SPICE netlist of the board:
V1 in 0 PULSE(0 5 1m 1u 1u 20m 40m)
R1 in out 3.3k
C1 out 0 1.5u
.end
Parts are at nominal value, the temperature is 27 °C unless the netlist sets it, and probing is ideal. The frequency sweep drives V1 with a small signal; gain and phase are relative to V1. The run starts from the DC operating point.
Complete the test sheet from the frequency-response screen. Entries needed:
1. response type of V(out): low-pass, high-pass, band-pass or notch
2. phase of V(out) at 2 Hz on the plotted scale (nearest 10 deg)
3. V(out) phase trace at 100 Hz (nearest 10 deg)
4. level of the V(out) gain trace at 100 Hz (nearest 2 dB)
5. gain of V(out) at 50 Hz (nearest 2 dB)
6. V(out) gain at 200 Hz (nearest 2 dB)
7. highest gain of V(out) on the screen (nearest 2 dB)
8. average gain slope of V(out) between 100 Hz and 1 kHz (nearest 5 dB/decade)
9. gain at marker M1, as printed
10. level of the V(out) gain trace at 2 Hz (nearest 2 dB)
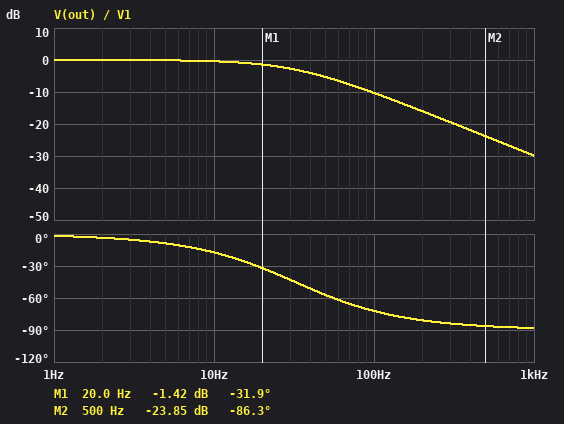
low-pass
0 deg
-70 deg
-10 dB
-6 dB
-16 dB
0 dB
-20 dB/decade
-1.42 dB
0 dB
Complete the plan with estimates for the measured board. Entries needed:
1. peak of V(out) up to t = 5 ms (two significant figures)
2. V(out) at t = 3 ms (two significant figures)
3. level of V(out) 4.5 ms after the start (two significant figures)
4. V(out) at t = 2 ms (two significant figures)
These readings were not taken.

2.8 V
1.7 V
2.5 V
910 mV
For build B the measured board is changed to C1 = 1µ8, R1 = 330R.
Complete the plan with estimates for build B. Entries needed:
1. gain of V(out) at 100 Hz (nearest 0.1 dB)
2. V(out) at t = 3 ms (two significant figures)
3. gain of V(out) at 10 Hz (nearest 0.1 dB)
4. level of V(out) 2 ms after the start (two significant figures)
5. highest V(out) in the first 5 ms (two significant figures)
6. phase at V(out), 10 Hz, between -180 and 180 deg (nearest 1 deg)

-0.6 dB
4.8 V
0 dB
4.1 V
5.0 V
-2 deg
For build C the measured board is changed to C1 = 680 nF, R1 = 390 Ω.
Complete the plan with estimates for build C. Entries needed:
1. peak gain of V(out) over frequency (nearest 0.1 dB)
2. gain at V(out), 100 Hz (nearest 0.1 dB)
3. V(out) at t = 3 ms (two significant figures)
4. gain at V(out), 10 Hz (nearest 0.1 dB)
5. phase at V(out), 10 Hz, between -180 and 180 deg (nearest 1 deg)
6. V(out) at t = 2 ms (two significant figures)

0 dB
-0.1 dB
5.0 V
0 dB
-1 deg
4.9 V
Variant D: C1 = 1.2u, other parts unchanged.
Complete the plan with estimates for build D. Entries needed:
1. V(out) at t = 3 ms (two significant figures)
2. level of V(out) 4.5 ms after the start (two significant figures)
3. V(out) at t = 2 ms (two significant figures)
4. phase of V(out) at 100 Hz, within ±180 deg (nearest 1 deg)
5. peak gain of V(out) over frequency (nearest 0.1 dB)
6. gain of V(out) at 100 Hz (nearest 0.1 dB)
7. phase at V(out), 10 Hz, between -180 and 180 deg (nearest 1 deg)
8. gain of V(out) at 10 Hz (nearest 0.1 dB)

2.0 V
2.9 V
1.1 V
-68 deg
0 dB
-8.6 dB
-14 deg
-0.3 dB
